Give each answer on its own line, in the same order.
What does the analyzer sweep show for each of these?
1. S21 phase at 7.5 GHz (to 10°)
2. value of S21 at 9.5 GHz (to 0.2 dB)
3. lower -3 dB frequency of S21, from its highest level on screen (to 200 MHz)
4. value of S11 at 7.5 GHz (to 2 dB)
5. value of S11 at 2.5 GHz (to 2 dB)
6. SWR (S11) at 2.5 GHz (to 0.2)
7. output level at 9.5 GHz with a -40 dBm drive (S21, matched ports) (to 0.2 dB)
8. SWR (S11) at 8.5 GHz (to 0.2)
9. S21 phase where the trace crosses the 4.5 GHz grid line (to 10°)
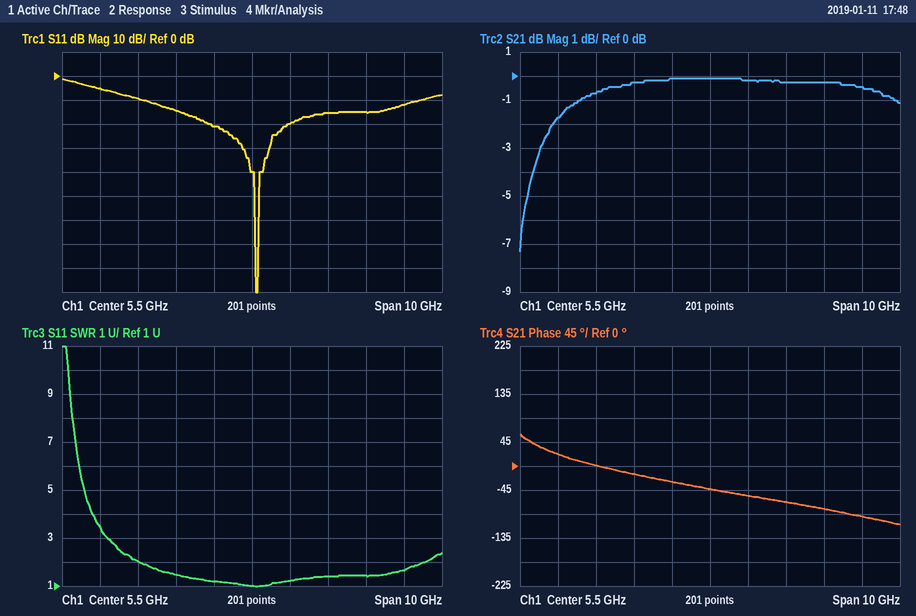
-70°
-0.4 dB
1.0 GHz
-16 dB
-10 dB
2.0
-40.4 dBm
1.4
-30°
